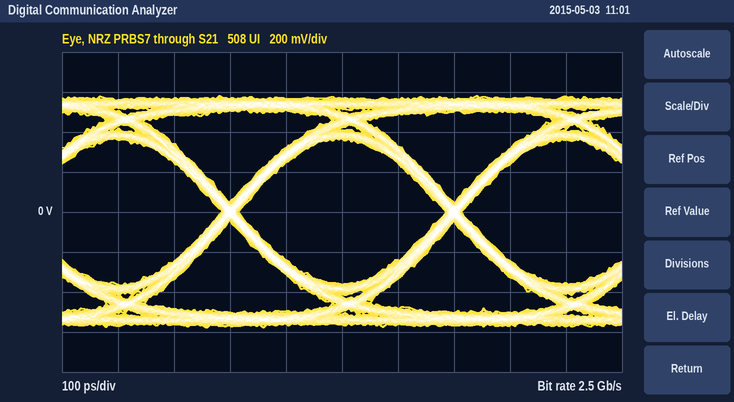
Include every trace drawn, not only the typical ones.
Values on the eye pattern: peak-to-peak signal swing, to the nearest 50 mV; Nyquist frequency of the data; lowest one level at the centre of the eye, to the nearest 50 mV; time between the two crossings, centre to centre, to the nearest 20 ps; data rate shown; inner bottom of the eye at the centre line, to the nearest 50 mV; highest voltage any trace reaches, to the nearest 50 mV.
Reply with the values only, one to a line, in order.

1.15 V
1.25 GHz
350 mV
400 ps
2.5 Gb/s
-350 mV
600 mV
